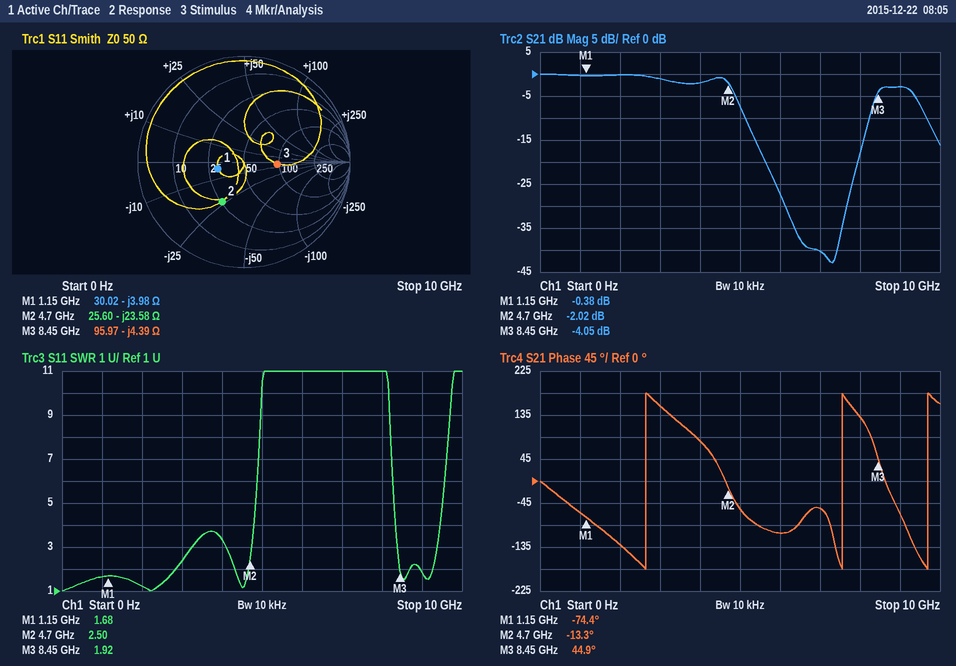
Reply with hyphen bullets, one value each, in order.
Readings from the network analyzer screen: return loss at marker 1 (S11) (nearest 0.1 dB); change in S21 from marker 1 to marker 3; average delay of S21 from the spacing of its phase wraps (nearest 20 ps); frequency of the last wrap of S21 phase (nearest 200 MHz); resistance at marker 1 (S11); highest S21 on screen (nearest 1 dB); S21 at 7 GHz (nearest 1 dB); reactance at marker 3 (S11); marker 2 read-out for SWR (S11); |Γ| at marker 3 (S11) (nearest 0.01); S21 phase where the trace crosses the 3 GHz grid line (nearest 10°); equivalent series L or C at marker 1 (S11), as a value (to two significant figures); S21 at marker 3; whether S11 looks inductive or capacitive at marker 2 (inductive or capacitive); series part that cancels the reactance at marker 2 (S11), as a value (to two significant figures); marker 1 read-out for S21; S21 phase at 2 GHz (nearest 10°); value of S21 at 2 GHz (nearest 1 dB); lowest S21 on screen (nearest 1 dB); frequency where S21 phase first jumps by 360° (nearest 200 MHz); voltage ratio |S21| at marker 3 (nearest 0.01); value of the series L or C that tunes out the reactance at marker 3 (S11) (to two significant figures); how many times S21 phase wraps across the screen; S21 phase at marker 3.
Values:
- 11.9 dB
- -3.67 dB
- 280 ps
- 9.6 GHz
- 30.02 Ω
- 0 dB
- -40 dB
- -4.39 Ω
- 2.50
- 0.32
- 150°
- 35 pF
- -4.05 dB
- capacitive
- 800 pH
- -0.38 dB
- -130°
- 0 dB
- -43 dB
- 2.6 GHz
- 0.63
- 83 pH
- 3
- 44.9°
